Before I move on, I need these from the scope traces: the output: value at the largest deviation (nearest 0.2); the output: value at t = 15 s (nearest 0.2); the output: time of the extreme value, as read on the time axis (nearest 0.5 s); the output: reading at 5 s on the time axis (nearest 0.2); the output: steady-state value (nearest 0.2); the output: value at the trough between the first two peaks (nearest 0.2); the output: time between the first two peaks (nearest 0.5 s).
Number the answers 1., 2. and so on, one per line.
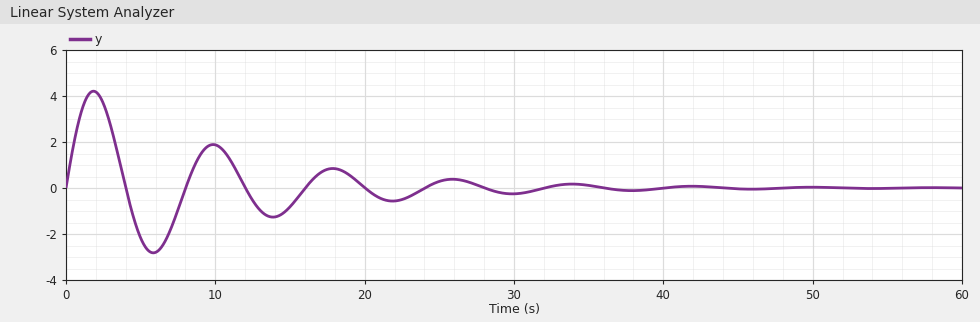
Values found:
1. 4.2
2. -0.8
3. 2.0 s
4. -2.2
5. 0.0
6. -2.8
7. 8.0 s
